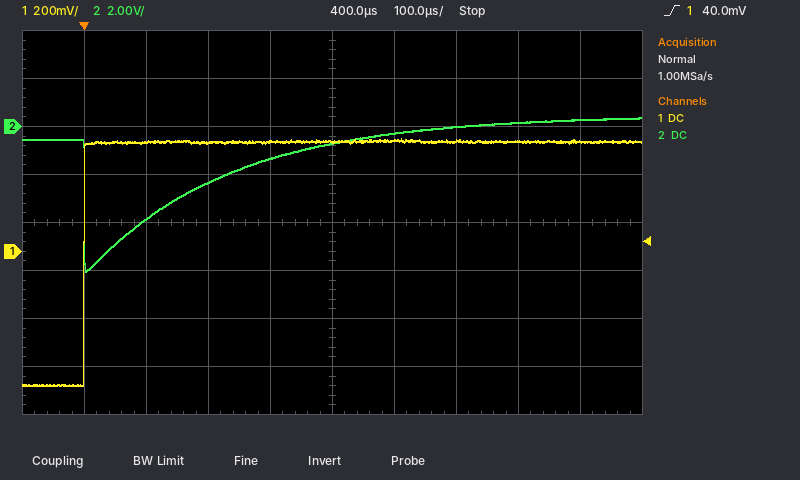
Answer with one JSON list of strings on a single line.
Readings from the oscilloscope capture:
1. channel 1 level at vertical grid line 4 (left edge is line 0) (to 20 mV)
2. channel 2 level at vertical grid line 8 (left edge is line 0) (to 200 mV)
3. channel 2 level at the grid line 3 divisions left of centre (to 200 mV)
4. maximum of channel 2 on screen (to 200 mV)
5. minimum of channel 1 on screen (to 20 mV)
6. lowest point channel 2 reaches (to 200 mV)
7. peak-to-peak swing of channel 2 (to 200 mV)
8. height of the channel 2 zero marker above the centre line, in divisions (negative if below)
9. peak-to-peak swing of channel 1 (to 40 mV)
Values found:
["460 mV", "200 mV", "-3.8 V", "400 mV", "-560 mV", "-6.0 V", "6.4 V", "+2.0 div", "1.04 V"]
